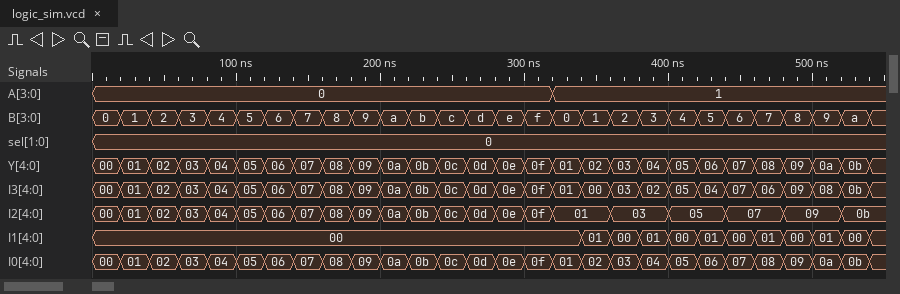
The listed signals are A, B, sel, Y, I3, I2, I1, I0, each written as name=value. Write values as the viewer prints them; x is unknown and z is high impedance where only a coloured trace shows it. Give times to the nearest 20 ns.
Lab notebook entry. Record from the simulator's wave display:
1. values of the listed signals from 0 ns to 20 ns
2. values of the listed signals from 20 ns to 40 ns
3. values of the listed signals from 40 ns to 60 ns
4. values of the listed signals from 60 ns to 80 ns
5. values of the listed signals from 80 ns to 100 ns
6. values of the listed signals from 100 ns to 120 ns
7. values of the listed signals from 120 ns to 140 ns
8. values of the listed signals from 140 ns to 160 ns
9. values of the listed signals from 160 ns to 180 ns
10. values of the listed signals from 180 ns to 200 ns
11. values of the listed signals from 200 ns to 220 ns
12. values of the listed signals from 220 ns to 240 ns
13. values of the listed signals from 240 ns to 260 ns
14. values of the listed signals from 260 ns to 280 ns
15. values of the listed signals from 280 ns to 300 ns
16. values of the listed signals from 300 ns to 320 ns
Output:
A=0, B=0, sel=0, Y=00, I3=00, I2=00, I1=00, I0=00
A=0, B=1, sel=0, Y=01, I3=01, I2=01, I1=00, I0=01
A=0, B=2, sel=0, Y=02, I3=02, I2=02, I1=00, I0=02
A=0, B=3, sel=0, Y=03, I3=03, I2=03, I1=00, I0=03
A=0, B=4, sel=0, Y=04, I3=04, I2=04, I1=00, I0=04
A=0, B=5, sel=0, Y=05, I3=05, I2=05, I1=00, I0=05
A=0, B=6, sel=0, Y=06, I3=06, I2=06, I1=00, I0=06
A=0, B=7, sel=0, Y=07, I3=07, I2=07, I1=00, I0=07
A=0, B=8, sel=0, Y=08, I3=08, I2=08, I1=00, I0=08
A=0, B=9, sel=0, Y=09, I3=09, I2=09, I1=00, I0=09
A=0, B=a, sel=0, Y=0a, I3=0a, I2=0a, I1=00, I0=0a
A=0, B=b, sel=0, Y=0b, I3=0b, I2=0b, I1=00, I0=0b
A=0, B=c, sel=0, Y=0c, I3=0c, I2=0c, I1=00, I0=0c
A=0, B=d, sel=0, Y=0d, I3=0d, I2=0d, I1=00, I0=0d
A=0, B=e, sel=0, Y=0e, I3=0e, I2=0e, I1=00, I0=0e
A=0, B=f, sel=0, Y=0f, I3=0f, I2=0f, I1=00, I0=0f
